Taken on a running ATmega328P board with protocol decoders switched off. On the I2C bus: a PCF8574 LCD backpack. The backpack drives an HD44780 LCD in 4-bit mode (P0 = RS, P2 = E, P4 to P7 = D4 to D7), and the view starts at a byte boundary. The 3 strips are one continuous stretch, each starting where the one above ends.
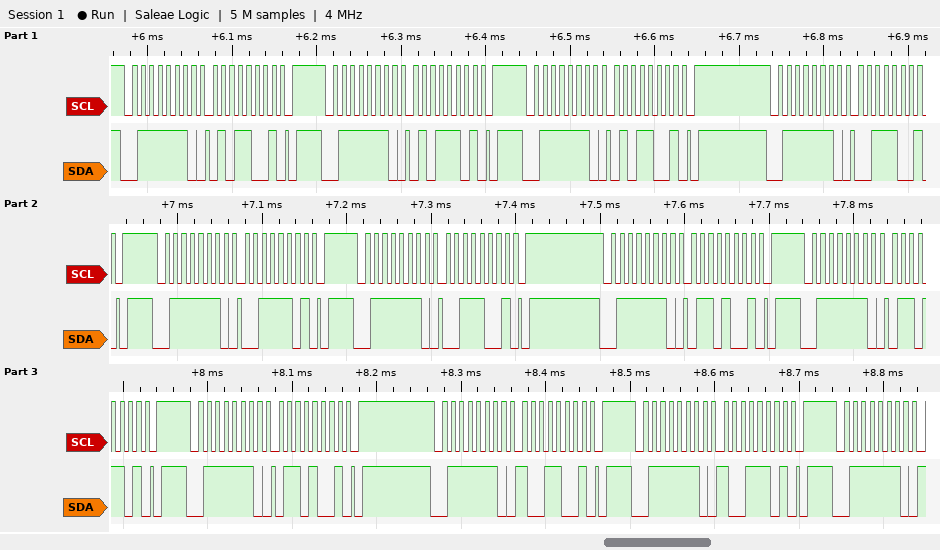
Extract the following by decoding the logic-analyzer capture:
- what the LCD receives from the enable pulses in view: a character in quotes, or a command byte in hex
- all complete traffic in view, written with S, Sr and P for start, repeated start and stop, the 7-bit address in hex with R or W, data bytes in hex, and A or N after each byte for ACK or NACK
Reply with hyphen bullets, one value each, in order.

- 'S'
- S 3FW A 59 A P S 3FW A 5D A P S 3FW A 59 A P S 3FW A 39 A P S 3FW A 3D A P S 3FW A 39 A P S 3FW A 69 A P S 3FW A 6D A P S 3FW A 69 A P S 3FW A 99 A P S 3FW A 9D A P S 3FW A
